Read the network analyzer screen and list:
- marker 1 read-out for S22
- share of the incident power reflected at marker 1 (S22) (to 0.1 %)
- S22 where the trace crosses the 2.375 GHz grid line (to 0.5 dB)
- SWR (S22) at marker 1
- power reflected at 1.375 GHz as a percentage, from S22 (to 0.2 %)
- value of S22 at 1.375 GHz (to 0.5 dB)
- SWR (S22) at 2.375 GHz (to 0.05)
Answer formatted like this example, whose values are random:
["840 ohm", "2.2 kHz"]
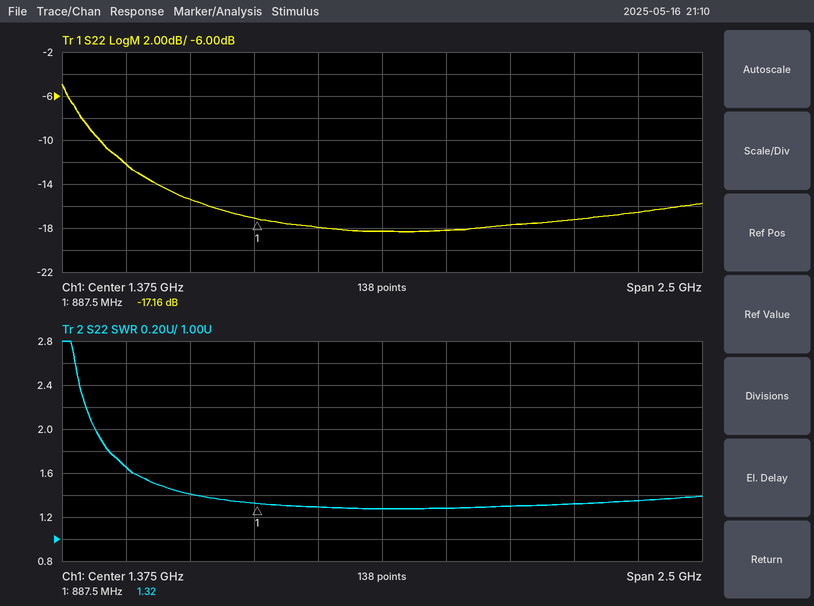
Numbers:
["-17.16 dB", "1.9 %", "-16.5 dB", "1.32", "1.4 %", "-18.5 dB", "1.35"]
